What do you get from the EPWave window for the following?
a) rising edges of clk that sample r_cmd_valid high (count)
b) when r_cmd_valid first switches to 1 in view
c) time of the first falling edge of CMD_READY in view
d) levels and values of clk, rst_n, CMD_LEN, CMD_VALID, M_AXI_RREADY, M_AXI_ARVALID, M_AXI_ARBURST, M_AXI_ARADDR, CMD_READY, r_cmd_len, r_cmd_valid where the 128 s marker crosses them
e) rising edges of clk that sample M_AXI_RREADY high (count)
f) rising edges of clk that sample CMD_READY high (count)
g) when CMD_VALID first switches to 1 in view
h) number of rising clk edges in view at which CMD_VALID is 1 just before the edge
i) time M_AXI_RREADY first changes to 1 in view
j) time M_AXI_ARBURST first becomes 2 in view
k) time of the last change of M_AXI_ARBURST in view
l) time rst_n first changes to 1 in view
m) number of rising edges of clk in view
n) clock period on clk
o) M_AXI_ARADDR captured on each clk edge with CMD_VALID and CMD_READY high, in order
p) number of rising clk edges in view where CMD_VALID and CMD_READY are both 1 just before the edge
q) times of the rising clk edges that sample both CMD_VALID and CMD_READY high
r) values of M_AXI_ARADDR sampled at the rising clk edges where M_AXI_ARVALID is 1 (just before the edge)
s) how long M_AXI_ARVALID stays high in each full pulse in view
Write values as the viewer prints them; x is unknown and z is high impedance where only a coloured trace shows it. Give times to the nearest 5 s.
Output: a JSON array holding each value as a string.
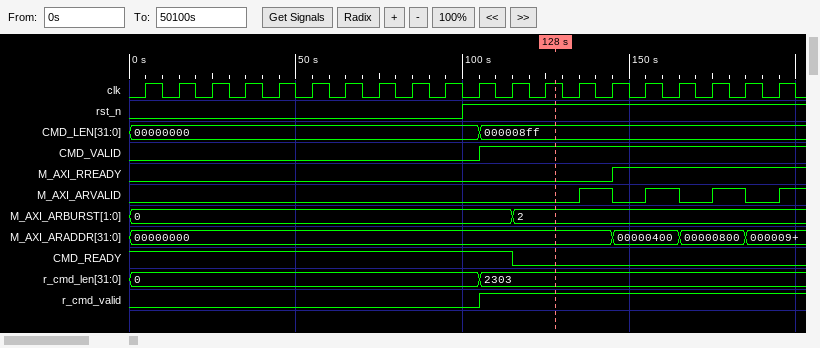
["9", "105 s", "115 s", "clk=1, rst_n=1, CMD_LEN=000008ff, CMD_VALID=1, M_AXI_RREADY=0, M_AXI_ARVALID=0, M_AXI_ARBURST=2, M_AXI_ARADDR=00000000, CMD_READY=0, r_cmd_len=2303, r_cmd_valid=1", "5", "12", "105 s", "9", "145 s", "115 s", "115 s", "100 s", "20", "10 s", "00000000", "1", "115 s", "00000000, 00000400, 00000800", "10 s, 10 s, 10 s"]
